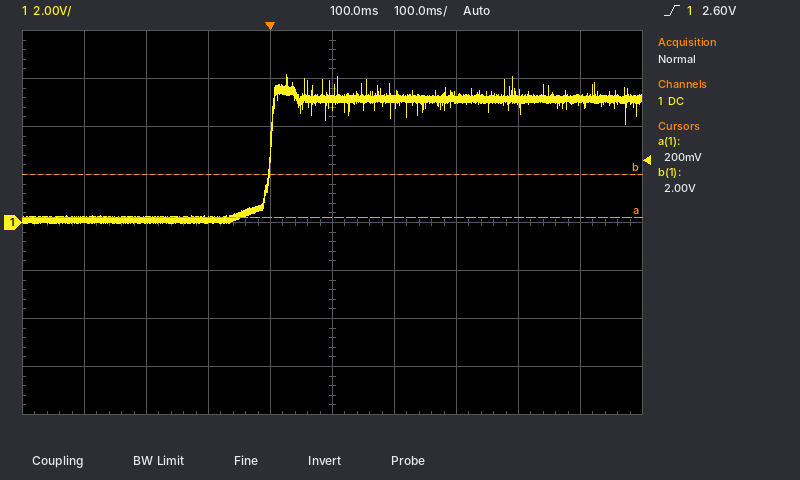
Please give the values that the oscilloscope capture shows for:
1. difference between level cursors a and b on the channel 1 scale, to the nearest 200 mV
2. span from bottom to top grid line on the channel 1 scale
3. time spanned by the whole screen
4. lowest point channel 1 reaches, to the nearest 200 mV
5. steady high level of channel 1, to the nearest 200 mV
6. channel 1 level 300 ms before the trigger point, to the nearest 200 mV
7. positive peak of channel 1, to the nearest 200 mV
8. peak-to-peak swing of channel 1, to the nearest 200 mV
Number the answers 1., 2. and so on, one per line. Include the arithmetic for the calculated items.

1. 1.8 V
2. 16 V
3. 1 s
4. 0.0 V
5. 5.2 V
6. 200 mV
7. 6.2 V
8. 6.2 V − (0.0 V) = 6.2 V
